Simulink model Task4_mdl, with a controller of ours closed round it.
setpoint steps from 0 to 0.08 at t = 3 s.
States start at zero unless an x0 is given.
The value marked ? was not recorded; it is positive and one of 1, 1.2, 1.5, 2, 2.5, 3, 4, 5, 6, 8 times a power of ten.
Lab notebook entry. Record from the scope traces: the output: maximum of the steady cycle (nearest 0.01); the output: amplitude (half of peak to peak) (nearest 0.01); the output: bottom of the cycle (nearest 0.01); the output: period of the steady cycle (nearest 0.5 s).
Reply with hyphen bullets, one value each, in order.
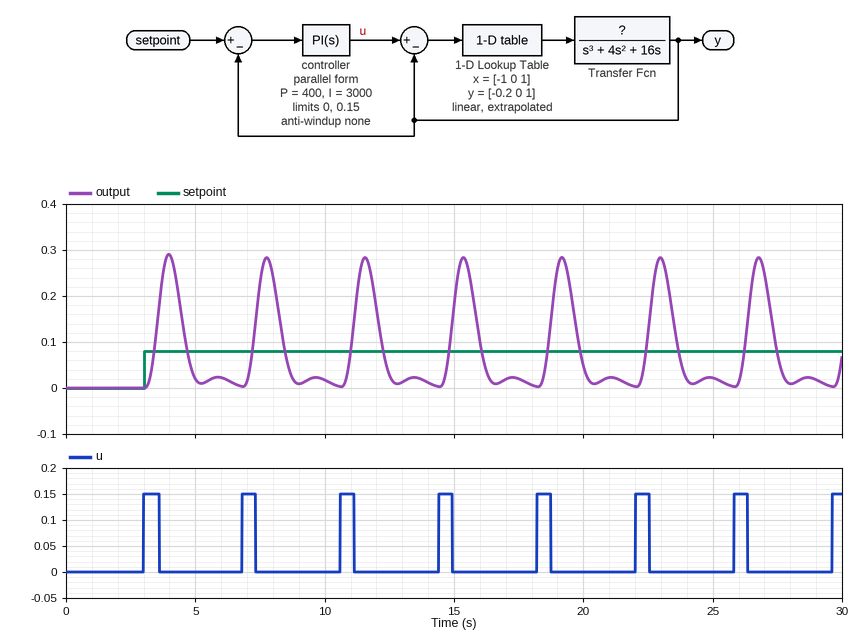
- 0.28
- 0.14
- 0.00
- 4.0 s
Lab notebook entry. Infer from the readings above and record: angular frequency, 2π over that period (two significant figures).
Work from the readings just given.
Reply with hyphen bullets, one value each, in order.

- 1.6 rad/s
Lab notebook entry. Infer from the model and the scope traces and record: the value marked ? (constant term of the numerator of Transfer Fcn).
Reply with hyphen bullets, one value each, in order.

- 80
